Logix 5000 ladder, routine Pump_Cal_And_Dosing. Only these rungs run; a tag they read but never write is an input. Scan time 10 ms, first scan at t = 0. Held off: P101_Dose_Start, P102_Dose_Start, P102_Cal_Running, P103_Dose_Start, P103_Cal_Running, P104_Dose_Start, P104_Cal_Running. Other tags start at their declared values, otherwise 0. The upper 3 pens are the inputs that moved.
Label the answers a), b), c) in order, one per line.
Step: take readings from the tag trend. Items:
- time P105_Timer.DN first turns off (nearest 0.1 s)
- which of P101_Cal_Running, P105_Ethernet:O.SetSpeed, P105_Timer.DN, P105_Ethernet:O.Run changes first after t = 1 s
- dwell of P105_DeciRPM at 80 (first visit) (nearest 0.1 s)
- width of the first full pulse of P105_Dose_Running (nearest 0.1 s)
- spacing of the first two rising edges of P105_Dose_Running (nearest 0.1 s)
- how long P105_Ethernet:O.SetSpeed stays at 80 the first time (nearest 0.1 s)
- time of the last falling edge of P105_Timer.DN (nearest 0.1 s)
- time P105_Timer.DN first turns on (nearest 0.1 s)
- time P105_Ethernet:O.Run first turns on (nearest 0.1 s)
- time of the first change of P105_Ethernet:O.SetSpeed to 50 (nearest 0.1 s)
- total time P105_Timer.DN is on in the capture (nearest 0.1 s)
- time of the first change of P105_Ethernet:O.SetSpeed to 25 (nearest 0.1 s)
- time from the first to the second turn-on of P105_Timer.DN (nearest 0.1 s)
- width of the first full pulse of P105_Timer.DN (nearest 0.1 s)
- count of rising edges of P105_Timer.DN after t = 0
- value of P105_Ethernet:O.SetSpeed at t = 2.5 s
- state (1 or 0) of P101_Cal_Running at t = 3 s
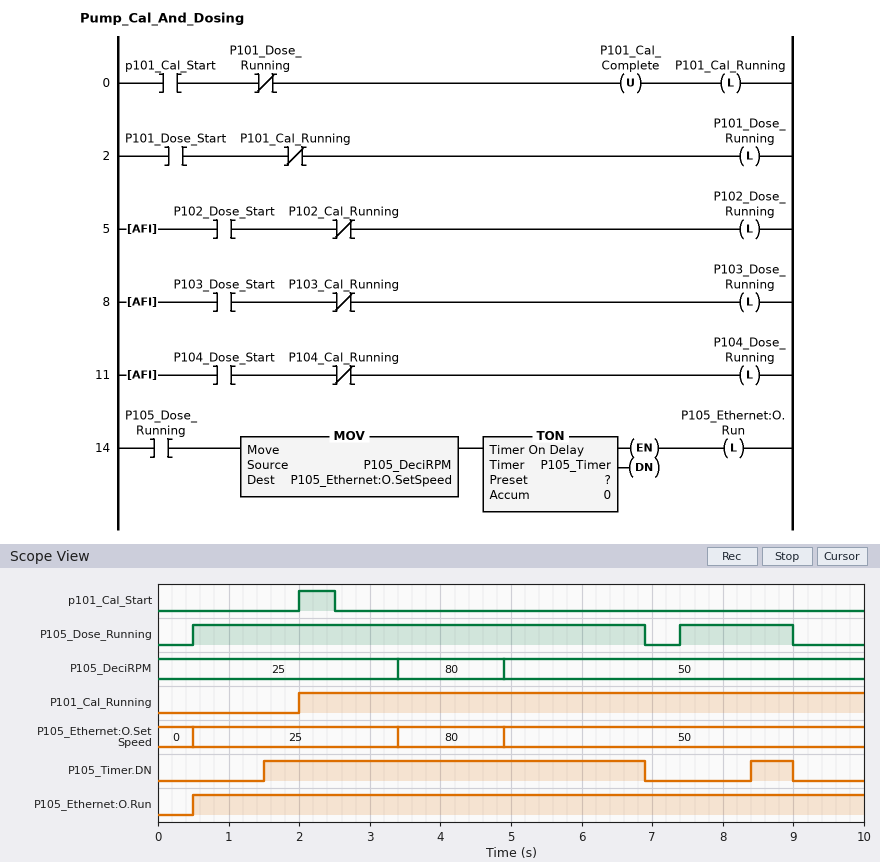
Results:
a) 6.9 s
b) P105_Timer.DN
c) 1.5 s
d) 6.4 s
e) 6.9 s
f) 1.5 s
g) 9.0 s
h) 1.5 s
i) 0.5 s
j) 4.9 s
k) 6.0 s
l) 0.5 s
m) 6.9 s
n) 5.4 s
o) 2
p) 25
q) 1
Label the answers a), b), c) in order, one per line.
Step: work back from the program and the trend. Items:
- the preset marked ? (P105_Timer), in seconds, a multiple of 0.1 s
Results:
a) 1.0 s
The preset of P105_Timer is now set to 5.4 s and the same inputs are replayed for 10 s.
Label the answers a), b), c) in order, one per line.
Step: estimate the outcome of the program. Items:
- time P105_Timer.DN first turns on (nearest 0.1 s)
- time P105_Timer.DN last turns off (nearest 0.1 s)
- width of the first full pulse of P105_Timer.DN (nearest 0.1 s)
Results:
a) 5.9 s
b) 6.9 s
c) 1.0 s
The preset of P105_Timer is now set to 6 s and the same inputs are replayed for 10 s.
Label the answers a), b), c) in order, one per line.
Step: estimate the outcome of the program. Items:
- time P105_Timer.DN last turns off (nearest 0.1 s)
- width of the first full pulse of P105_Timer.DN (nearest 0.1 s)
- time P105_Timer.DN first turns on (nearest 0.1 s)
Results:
a) 6.9 s
b) 0.4 s
c) 6.5 s
